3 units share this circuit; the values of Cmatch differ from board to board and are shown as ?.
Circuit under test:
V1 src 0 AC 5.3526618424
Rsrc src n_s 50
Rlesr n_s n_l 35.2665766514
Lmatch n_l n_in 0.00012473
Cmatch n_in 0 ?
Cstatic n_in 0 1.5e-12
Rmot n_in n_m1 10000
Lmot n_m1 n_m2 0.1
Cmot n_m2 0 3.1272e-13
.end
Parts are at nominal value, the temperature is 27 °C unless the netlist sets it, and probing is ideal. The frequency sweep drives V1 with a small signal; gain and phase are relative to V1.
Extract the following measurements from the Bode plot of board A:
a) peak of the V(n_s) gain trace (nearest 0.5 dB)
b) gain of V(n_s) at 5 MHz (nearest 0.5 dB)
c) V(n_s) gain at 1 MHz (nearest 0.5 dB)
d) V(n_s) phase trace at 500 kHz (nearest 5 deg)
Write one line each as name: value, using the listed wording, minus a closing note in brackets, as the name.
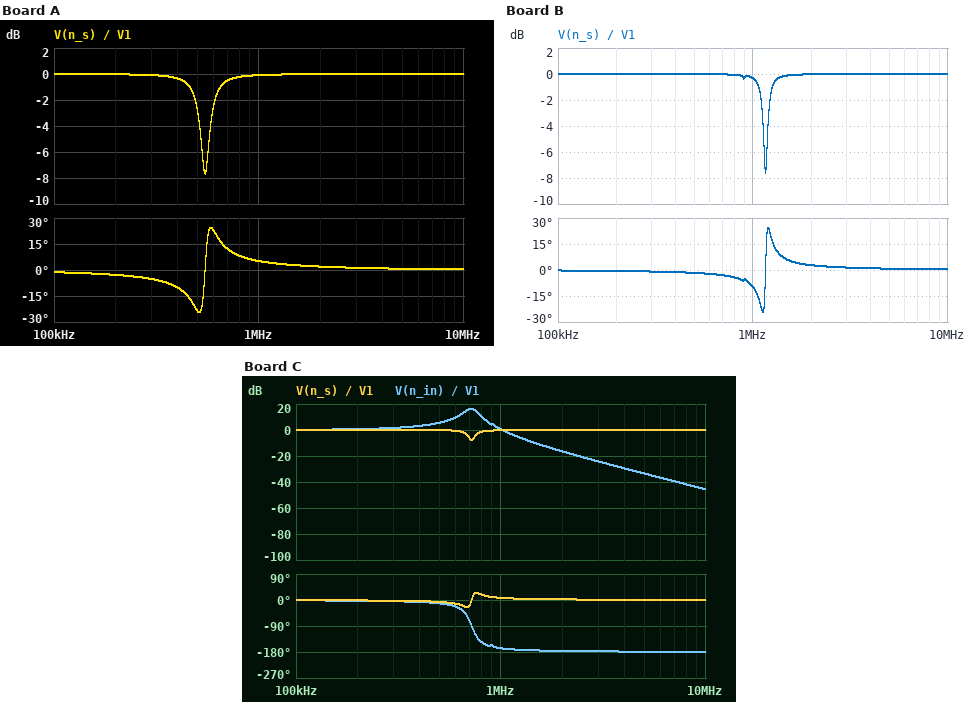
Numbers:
peak of the V(n_s) gain trace: 0 dB
gain of V(n_s) at 5 MHz: 0 dB
V(n_s) gain at 1 MHz: 0 dB
V(n_s) phase trace at 500 kHz: -25 deg
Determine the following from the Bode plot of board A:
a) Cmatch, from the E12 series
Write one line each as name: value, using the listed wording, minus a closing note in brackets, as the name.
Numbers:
Cmatch, from the E12 series: 680 pF
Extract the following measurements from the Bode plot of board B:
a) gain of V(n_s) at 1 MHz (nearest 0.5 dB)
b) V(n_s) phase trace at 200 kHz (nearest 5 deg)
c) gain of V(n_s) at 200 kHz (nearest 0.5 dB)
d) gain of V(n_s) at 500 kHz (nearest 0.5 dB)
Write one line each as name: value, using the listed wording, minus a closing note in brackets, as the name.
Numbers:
gain of V(n_s) at 1 MHz: -0.5 dB
V(n_s) phase trace at 200 kHz: 0 deg
gain of V(n_s) at 200 kHz: 0 dB
gain of V(n_s) at 500 kHz: 0 dB
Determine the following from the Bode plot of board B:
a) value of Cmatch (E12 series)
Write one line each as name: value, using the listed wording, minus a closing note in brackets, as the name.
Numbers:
value of Cmatch: 150 pF
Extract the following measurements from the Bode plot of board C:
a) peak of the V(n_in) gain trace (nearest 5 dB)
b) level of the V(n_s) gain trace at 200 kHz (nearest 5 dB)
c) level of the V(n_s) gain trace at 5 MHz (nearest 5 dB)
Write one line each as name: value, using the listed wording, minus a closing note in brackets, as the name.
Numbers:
peak of the V(n_in) gain trace: 15 dB
level of the V(n_s) gain trace at 200 kHz: 0 dB
level of the V(n_s) gain trace at 5 MHz: 0 dB
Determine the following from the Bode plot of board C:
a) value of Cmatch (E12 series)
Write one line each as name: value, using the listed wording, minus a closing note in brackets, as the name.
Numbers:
value of Cmatch: 390 pF
